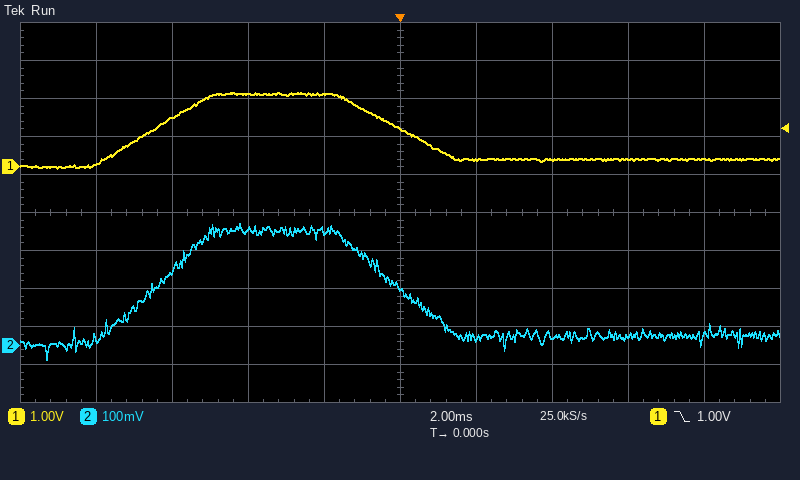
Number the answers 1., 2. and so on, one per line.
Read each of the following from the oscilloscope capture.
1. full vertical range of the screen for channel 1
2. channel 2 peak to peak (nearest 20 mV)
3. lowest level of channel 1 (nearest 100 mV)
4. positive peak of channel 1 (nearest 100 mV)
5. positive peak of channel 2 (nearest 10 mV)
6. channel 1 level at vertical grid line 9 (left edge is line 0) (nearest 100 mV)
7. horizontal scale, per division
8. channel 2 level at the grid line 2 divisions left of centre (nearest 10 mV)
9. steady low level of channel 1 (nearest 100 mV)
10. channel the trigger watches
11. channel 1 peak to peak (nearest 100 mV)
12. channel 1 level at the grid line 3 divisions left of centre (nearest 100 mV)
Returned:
1. 10 V
2. 360 mV
3. 0.0 V
4. 2.0 V
5. 320 mV
6. 200 mV
7. 2 ms
8. 300 mV
9. 200 mV
10. channel 1
11. 2.0 V
12. 1.3 V
